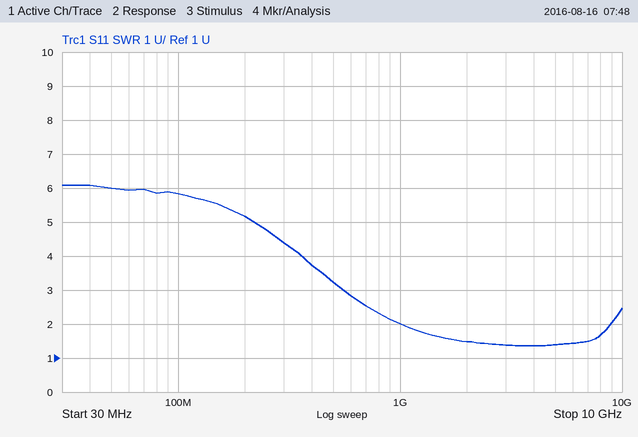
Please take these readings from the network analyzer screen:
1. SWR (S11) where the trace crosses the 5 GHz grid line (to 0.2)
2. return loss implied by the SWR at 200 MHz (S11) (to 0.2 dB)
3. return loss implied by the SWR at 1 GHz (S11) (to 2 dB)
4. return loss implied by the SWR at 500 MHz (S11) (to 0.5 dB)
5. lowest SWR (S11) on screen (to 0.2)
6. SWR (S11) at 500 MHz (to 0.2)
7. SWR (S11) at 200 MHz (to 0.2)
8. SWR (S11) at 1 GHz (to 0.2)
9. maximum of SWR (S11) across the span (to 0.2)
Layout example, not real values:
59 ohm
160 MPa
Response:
1.4
3.4 dB
10 dB
5.5 dB
1.4
3.2
5.2
2.0
6.0
